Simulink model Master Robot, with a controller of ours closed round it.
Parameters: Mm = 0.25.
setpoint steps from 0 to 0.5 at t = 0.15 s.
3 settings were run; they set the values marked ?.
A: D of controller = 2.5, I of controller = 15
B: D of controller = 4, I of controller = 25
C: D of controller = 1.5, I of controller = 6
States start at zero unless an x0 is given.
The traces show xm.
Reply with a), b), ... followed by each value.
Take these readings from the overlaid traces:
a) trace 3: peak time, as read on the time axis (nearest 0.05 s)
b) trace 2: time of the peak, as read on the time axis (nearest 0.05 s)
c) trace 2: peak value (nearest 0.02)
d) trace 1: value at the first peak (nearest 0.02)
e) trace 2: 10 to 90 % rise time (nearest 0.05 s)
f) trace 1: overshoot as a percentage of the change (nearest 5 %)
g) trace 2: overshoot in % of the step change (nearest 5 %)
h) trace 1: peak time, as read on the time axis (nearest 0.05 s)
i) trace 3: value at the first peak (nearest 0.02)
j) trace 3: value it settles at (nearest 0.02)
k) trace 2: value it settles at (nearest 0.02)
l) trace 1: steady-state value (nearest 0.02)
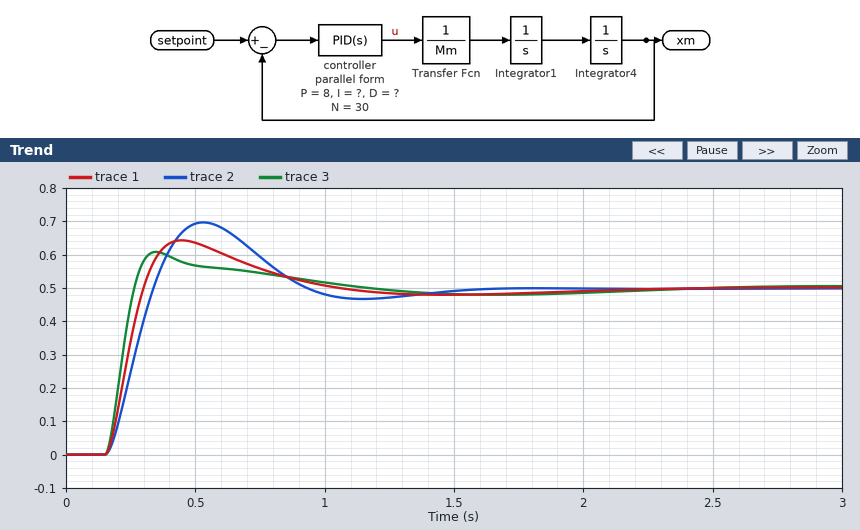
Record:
a) 0.35 s
b) 0.55 s
c) 0.70
d) 0.64
e) 0.15 s
f) 30 %
g) 40 %
h) 0.45 s
i) 0.60
j) 0.50
k) 0.50
l) 0.50
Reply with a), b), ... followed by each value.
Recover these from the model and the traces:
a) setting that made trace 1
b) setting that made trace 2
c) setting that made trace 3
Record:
a) A
b) C
c) B
